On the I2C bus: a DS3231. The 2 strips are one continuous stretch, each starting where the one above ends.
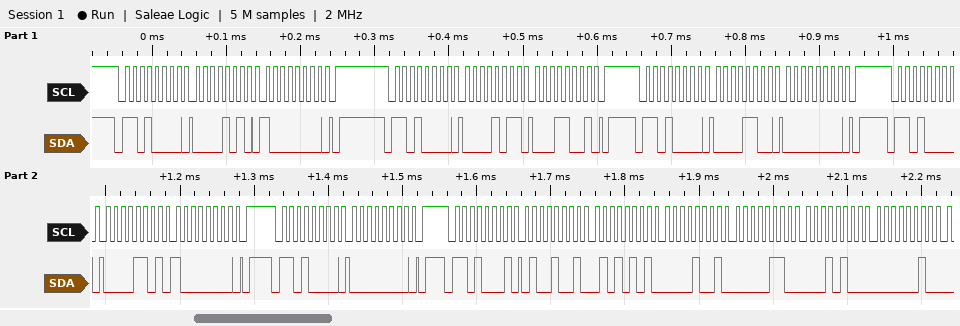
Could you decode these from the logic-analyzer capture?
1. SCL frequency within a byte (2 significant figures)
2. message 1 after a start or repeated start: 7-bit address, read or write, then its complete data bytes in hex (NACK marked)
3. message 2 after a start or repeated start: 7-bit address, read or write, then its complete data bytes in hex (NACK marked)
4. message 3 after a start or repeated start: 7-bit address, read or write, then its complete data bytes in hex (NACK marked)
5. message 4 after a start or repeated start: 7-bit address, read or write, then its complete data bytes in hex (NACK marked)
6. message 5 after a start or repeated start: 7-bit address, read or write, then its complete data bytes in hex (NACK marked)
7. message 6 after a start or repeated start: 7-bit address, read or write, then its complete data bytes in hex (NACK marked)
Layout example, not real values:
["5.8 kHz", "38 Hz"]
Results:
["100 kHz", "0x68 write: 0A 80", "0x68 write: 0B 19", "0x68 write: 0C 00", "0x68 write: 0D 80", "0x68 write: 00", "0x68 read: 49 55 09 06 14 02"]
